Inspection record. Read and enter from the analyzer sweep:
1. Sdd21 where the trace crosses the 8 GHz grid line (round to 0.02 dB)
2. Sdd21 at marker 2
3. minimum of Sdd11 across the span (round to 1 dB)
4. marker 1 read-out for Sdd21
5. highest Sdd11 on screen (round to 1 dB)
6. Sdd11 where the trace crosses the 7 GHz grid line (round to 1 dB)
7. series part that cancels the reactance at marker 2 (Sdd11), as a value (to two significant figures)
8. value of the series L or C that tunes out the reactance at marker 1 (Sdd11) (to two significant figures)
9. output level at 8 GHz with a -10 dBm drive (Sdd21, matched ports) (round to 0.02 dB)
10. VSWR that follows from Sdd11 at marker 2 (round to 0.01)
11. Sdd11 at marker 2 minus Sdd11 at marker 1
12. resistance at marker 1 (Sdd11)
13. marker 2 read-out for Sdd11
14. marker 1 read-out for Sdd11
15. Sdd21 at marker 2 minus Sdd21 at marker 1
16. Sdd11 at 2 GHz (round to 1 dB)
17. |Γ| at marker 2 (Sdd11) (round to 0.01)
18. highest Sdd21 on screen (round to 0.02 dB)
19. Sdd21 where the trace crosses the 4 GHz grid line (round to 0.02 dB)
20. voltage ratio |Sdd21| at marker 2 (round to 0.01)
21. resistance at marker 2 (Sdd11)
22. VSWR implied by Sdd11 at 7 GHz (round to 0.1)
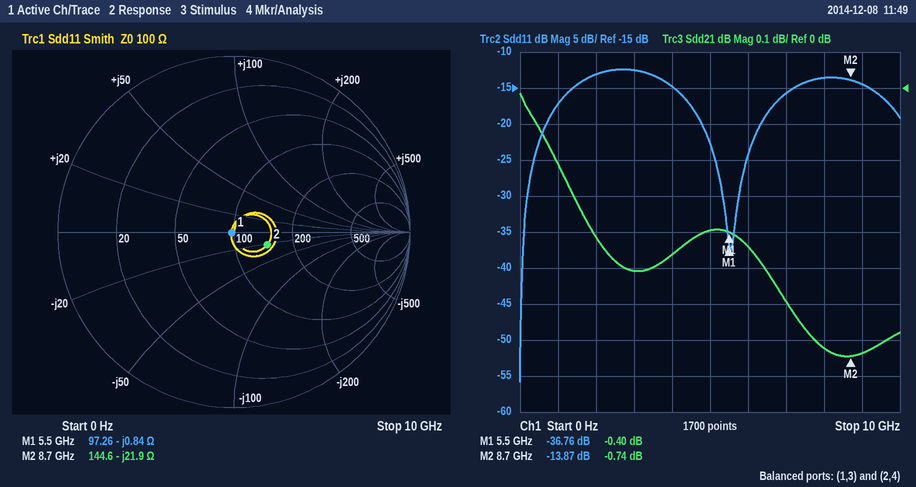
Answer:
-0.72 dB
-0.74 dB
-56 dB
-0.40 dB
-12 dB
-16 dB
400 pH
24 pH
-10.72 dBm
1.51
22.89 dB
97.26 Ω
-13.87 dB
-36.76 dB
-0.34 dB
-13 dB
0.20
-0.02 dB
-0.46 dB
0.92
144.6 Ω
1.4
